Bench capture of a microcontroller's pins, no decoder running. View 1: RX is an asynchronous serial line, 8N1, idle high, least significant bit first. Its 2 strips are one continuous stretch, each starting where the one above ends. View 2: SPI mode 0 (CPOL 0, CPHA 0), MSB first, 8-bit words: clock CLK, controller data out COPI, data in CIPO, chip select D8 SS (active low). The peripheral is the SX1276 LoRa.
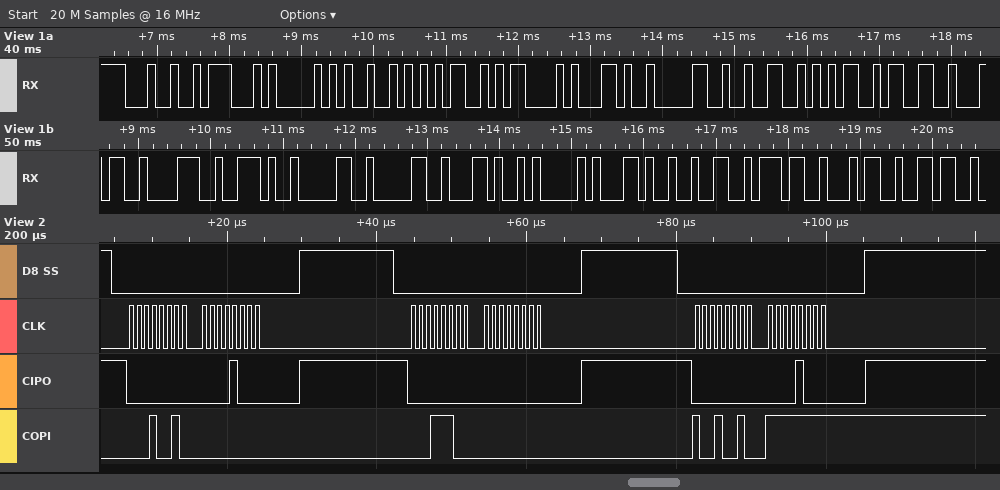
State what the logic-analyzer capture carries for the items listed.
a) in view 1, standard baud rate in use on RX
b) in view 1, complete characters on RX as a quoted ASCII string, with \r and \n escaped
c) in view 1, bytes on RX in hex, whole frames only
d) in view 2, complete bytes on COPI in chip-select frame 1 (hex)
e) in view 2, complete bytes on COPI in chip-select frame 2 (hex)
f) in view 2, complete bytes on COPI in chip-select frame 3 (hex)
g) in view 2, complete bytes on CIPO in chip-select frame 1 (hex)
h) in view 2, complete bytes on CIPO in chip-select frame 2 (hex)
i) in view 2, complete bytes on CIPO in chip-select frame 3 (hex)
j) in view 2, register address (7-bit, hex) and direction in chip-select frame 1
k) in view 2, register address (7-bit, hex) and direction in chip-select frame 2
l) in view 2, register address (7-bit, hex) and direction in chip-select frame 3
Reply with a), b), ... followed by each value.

a) 9600 baud
b) "$GPRMC,025348.00,A,2746"
c) 24 47 50 52 4D 43 2C 30 32 35 33 34 38 2E 30 30 2C 41 2C 32 37 34 36
d) 0x12 0x00
e) 0x1C 0x00
f) 0x92 0xFF
g) 0x00 0x08
h) 0x00 0x00
i) 0x00 0x08
j) 0x12 read
k) 0x1C read
l) 0x12 write
